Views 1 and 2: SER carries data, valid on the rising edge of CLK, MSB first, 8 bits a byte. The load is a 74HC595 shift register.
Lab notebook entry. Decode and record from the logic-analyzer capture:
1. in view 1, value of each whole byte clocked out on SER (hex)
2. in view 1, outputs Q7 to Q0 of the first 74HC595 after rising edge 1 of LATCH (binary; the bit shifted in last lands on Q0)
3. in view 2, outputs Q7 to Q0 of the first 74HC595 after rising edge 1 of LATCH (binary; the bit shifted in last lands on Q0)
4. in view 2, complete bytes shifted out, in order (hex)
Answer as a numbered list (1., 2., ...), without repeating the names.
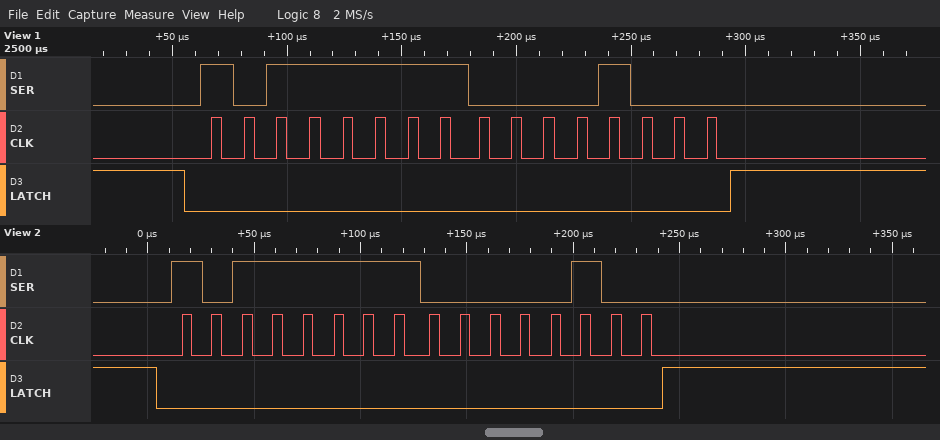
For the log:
1. BF 08
2. 00001000
3. 00000100
4. BF 04
